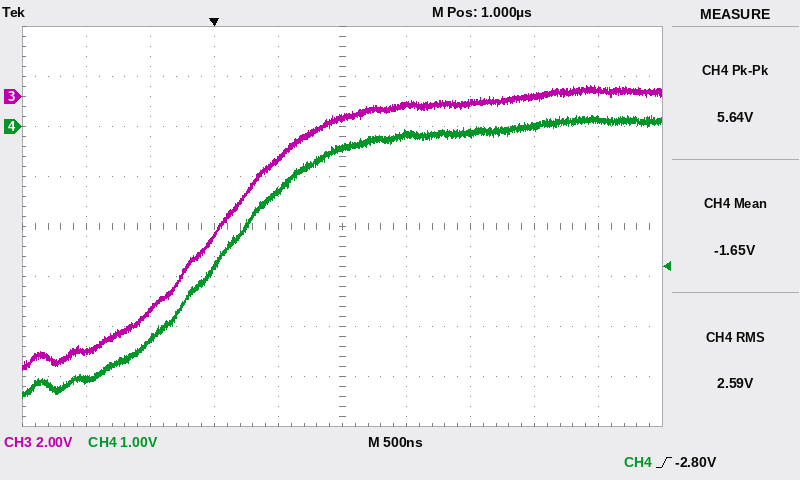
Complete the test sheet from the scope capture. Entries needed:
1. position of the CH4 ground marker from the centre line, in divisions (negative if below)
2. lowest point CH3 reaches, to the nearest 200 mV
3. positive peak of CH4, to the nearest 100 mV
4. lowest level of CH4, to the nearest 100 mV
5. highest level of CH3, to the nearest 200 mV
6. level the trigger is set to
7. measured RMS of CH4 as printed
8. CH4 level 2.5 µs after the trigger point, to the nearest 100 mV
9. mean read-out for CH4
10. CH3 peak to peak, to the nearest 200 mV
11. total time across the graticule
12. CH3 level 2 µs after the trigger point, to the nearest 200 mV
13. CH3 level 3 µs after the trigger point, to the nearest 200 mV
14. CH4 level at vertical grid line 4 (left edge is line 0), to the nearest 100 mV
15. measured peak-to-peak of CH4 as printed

+2.0 div
-11.0 V
200 mV
-5.4 V
400 mV
-2.80 V
2.59 V
0.0 V
-1.65 V
11.4 V
5 µs
-200 mV
200 mV
-1.3 V
5.64 V
